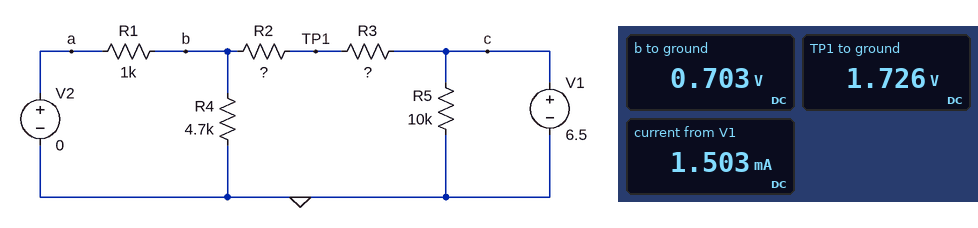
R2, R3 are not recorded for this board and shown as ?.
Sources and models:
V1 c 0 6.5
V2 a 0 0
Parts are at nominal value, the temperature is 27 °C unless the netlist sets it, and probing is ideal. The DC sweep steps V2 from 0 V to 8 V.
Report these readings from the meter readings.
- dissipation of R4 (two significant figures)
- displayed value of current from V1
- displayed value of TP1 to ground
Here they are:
110 µW
1.503 mA
1.726 V
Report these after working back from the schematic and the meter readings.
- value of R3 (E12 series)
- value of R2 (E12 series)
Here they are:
5.6 kΩ
1.2 kΩ
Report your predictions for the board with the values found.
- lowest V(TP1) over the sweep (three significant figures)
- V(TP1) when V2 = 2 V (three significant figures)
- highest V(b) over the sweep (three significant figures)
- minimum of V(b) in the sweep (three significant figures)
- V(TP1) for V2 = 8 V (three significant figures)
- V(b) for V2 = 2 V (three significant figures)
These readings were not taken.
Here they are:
1.73 V
2.94 V
6.59 V
703 mV
6.57 V
2.17 V
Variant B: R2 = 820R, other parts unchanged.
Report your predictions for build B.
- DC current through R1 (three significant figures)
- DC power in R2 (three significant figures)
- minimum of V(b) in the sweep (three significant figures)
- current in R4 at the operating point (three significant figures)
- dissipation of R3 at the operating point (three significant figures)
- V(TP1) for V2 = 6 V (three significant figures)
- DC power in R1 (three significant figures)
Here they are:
740 µA
660 µW
740 mV
157 µA
4.51 mW
5.30 V
547 µW
